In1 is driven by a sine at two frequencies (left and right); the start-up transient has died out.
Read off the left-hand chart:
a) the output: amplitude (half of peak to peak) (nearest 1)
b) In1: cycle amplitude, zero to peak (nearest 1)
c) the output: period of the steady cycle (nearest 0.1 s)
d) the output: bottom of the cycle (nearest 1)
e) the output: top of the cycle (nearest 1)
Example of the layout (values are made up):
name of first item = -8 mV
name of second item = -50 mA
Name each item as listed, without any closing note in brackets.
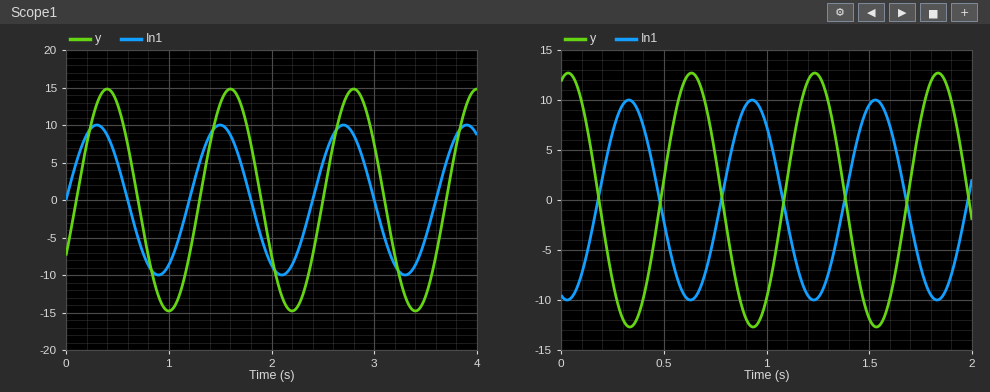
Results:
the output: amplitude (half of peak to peak) = 15
In1: cycle amplitude, zero to peak = 10
the output: period of the steady cycle = 1.2 s
the output: bottom of the cycle = -15
the output: top of the cycle = 15
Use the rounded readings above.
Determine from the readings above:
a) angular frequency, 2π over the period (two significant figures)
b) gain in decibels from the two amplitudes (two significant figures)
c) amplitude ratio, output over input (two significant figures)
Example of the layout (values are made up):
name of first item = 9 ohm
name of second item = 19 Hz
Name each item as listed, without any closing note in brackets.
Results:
angular frequency, 2π over the period = 5.2 rad/s
gain in decibels from the two amplitudes = 3.5 dB
amplitude ratio, output over input = 1.5
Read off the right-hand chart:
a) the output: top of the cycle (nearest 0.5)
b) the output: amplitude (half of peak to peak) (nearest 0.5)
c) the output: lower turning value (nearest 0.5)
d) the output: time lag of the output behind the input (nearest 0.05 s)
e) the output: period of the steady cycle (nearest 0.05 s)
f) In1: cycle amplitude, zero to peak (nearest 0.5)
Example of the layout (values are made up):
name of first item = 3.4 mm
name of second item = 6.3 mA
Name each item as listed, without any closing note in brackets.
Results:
the output: top of the cycle = 12.5
the output: amplitude (half of peak to peak) = 12.5
the output: lower turning value = -12.5
the output: time lag of the output behind the input = 0.30 s
the output: period of the steady cycle = 0.60 s
In1: cycle amplitude, zero to peak = 10.0
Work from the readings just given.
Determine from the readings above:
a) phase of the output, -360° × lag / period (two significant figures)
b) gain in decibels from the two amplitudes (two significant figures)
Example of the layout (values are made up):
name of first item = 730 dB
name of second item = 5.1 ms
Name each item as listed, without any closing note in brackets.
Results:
phase of the output, -360° × lag / period = -180°
gain in decibels from the two amplitudes = 1.9 dB
